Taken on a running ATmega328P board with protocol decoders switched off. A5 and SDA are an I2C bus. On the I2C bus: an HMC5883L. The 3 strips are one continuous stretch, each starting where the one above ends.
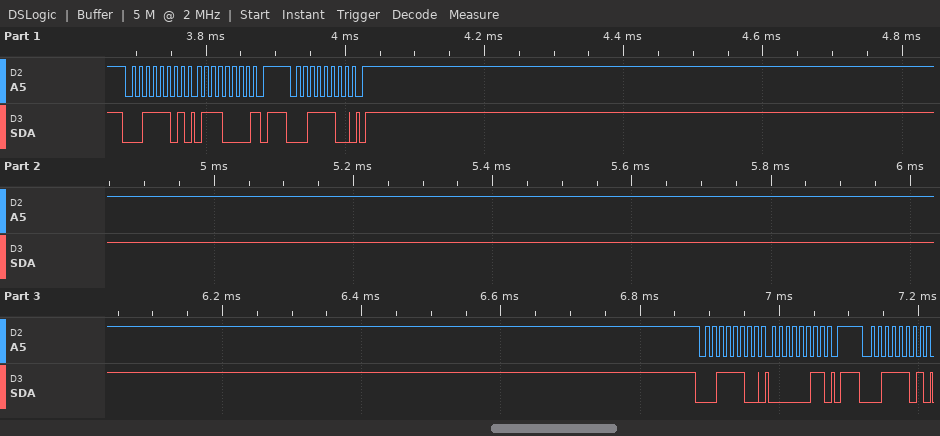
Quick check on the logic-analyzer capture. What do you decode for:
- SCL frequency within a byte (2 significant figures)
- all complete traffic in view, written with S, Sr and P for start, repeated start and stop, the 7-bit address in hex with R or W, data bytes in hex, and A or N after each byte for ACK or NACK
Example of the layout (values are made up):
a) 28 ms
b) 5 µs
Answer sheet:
a) 100 kHz
b) S 1ER A 70 N P S 1EW A P S 1EW A 03 A P S 1ER A
